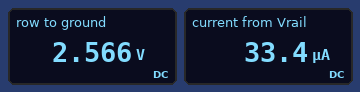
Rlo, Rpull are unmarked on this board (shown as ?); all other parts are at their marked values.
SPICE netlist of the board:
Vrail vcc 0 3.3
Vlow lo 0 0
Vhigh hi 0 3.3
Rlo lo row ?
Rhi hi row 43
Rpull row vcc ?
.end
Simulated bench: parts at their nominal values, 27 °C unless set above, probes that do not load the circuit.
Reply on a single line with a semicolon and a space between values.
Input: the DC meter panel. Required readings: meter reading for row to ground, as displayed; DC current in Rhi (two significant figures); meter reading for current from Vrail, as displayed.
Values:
2.566 V; 17 mA; 33.4 µA
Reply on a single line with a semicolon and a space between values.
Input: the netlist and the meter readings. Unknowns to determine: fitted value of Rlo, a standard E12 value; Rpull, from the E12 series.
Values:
150 Ω; 22 kΩ
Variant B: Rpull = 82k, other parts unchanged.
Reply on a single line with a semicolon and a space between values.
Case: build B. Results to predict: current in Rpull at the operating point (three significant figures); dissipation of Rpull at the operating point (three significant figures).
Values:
8.96 µA; 6.59 µW
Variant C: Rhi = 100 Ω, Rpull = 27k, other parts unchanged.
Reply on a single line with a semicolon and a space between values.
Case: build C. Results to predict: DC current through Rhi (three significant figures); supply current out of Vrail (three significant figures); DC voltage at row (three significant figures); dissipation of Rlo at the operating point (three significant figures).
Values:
13.2 mA; 48.8 µA; 1.98 V; 26.2 mW
